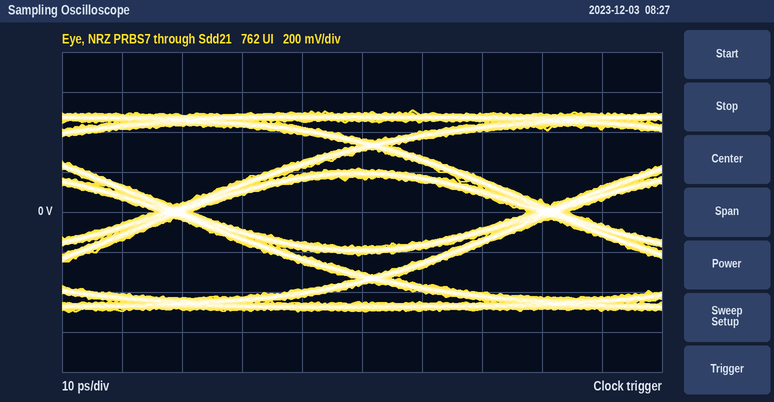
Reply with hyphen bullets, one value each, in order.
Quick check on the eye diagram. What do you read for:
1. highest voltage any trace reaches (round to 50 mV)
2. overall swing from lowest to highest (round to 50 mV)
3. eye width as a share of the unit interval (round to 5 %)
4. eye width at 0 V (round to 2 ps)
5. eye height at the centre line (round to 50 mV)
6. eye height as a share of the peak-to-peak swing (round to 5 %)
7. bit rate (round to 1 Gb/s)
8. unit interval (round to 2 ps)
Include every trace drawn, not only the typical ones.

- 500 mV
- 1.00 V
- 90 %
- 56 ps
- 350 mV
- 35 %
- 16 Gb/s
- 62 ps
